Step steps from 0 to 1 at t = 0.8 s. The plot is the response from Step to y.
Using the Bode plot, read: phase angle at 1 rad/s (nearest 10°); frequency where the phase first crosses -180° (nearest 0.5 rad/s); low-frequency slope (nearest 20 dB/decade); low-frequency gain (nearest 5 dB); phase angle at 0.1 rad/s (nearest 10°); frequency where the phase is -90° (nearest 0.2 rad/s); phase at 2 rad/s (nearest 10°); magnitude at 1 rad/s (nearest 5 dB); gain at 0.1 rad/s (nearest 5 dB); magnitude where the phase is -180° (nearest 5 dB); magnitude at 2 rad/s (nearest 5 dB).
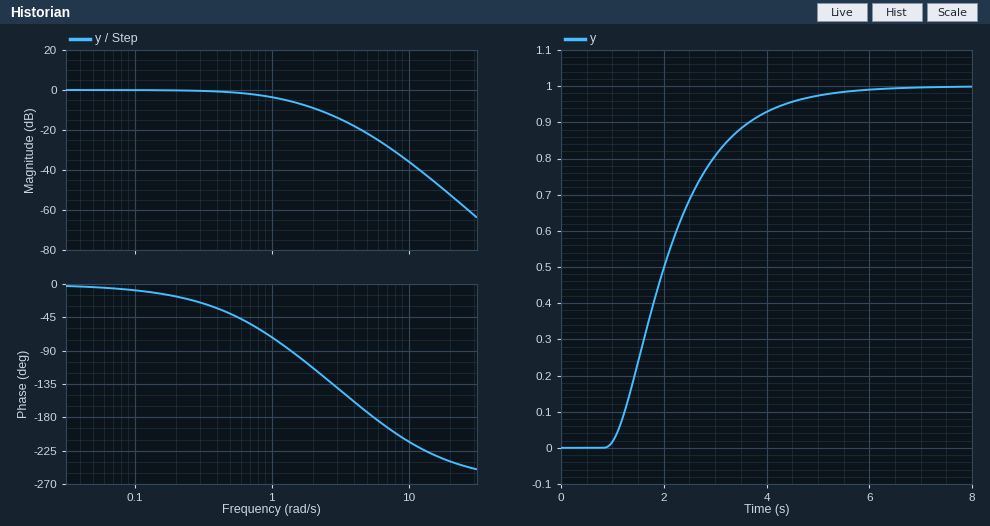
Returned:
-70°
5.5 rad/s
0 dB/decade
0 dB
-10°
1.4 rad/s
-110°
-5 dB
0 dB
-25 dB
-10 dB
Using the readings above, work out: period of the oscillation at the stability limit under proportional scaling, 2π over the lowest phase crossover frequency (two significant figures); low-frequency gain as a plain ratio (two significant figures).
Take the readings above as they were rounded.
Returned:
1.1 s
1.0
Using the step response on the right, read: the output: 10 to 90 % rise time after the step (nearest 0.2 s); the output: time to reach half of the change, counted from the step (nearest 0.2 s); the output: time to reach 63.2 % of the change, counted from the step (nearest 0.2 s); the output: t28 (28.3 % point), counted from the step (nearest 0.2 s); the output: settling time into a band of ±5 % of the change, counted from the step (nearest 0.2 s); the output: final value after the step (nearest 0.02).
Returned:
2.4 s
1.2 s
1.6 s
0.8 s
3.6 s
1.00
